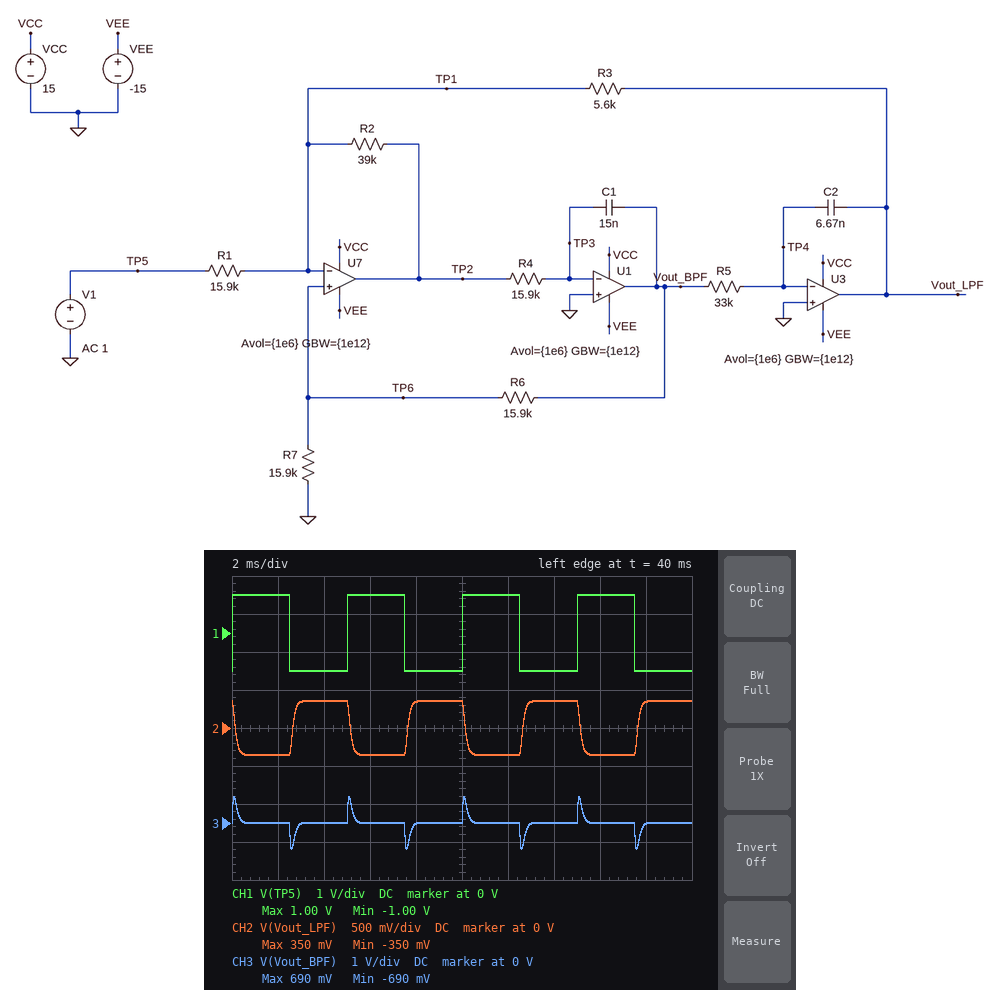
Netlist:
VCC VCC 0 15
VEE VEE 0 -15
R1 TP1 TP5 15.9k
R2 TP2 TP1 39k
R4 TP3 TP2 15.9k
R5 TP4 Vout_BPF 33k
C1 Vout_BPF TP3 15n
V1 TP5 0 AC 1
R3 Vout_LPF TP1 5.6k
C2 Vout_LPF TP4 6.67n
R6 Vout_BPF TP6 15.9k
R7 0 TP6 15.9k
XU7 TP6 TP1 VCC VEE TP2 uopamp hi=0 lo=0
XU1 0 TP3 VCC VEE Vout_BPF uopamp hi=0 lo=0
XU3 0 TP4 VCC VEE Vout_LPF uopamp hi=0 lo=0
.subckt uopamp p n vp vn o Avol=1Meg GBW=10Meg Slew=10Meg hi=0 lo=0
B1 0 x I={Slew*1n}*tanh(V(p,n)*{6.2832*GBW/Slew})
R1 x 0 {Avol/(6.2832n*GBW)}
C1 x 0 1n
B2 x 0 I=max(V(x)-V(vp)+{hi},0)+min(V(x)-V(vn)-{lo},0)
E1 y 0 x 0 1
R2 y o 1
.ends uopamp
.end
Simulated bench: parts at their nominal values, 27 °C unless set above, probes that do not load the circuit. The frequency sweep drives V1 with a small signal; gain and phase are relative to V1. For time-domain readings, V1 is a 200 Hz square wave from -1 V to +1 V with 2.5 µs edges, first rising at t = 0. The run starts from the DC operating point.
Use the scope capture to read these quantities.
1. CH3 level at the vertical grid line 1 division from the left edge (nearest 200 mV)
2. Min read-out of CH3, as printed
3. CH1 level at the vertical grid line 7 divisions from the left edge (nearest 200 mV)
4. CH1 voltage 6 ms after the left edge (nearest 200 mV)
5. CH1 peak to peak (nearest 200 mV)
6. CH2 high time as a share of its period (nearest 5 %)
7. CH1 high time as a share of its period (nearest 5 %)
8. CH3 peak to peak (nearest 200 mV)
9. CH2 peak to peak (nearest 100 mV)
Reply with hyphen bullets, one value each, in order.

- 0 V
- -690 mV
- -1.0 V
- 1.0 V
- 2.0 V
- 50 %
- 50 %
- 1.4 V
- 700 mV
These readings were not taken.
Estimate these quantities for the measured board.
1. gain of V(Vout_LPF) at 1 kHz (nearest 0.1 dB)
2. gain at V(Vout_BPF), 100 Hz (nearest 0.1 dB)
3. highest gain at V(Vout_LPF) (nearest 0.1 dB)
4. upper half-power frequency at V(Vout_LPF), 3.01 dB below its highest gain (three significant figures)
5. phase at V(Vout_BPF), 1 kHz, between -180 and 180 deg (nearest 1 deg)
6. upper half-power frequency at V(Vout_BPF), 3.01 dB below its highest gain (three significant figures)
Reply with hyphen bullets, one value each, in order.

- -11.0 dB
- -26.3 dB
- -9.1 dB
- 1.27 kHz
- 34 deg
- 4.27 kHz
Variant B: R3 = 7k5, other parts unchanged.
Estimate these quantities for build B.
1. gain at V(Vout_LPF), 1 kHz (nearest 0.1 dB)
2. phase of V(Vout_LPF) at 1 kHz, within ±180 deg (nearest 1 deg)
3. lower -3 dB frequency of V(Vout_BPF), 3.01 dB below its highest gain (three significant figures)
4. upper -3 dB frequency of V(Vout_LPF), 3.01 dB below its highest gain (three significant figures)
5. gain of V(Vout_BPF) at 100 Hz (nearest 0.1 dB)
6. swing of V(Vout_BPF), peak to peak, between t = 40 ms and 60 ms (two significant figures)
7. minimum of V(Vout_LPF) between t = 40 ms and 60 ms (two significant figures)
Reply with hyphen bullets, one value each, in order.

- -8.8 dB
- 118 deg
- 700 Hz
- 1.16 kHz
- -23.7 dB
- 1.6 V
- -470 mV
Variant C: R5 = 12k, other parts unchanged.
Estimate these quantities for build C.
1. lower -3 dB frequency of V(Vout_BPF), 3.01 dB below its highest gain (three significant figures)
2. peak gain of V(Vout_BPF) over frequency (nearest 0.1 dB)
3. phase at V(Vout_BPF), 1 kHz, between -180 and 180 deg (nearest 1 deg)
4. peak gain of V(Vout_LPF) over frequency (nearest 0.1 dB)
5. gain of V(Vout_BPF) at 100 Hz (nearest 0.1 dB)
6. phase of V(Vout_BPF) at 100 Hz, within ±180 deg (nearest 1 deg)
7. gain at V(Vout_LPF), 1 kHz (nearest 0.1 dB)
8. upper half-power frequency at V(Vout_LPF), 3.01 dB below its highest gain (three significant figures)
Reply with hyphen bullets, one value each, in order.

- 1.77 kHz
- -6.5 dB
- 67 deg
- -8.5 dB
- -35.0 dB
- 88 deg
- -8.8 dB
- 3.45 kHz
